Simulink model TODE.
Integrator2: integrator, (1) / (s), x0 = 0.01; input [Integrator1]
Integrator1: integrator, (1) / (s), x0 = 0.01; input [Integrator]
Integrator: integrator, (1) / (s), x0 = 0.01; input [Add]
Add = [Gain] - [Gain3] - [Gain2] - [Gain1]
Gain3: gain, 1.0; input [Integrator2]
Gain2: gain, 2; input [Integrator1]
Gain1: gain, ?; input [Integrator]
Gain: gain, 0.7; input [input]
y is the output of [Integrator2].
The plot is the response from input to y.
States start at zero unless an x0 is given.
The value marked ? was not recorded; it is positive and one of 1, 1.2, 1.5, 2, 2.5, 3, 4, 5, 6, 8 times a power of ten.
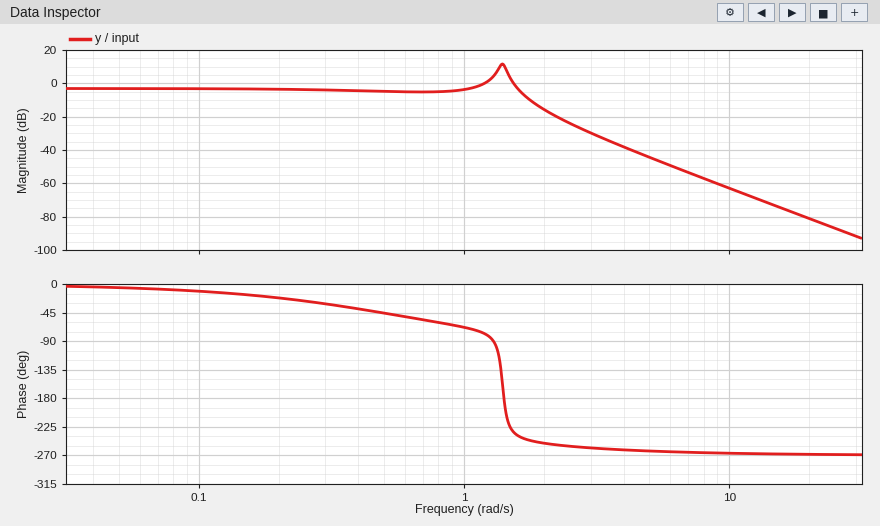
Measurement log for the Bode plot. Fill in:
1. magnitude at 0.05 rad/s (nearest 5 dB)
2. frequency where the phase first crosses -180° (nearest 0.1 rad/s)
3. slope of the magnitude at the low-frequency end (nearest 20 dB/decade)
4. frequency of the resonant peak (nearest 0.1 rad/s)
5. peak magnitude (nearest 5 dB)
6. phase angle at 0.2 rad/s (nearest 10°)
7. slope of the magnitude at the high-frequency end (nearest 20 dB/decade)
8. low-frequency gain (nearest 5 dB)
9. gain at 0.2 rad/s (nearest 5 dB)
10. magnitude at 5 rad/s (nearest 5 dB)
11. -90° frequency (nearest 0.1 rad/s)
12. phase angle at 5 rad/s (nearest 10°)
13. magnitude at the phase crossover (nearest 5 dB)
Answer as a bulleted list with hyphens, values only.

- -5 dB
- 1.4 rad/s
- 0 dB/decade
- 1.4 rad/s
- 10 dB
- -20°
- -60 dB/decade
- -5 dB
- -5 dB
- -45 dB
- 1.3 rad/s
- -260°
- 10 dB
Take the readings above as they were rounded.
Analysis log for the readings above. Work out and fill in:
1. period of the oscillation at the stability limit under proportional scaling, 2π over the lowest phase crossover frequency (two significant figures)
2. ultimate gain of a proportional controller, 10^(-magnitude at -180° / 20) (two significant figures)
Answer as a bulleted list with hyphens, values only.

- 4.5 s
- 0.32
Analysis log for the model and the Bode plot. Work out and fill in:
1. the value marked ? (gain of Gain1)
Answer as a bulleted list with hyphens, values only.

- 0.6
